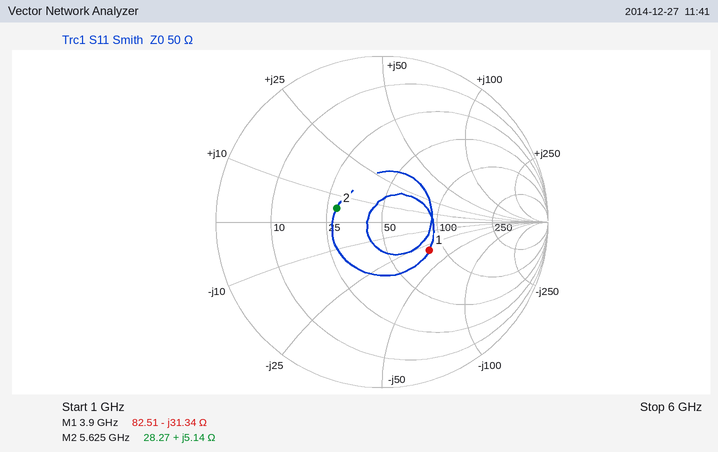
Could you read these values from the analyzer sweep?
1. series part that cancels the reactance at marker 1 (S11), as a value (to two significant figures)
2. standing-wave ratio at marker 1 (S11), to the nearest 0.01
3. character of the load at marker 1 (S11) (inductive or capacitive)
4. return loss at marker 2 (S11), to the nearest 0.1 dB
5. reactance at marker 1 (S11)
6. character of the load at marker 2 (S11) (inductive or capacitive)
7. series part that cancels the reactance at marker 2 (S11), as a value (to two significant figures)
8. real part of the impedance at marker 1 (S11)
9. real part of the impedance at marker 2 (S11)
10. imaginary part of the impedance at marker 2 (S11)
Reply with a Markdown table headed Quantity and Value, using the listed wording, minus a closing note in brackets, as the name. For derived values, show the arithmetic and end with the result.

| Quantity | Value |
|---|---|
| series part that cancels the reactance at marker 1 (S11), as a value | L = 31.34 Ω/(2π × 3.9 GHz) ≈ 1.3 nH |
| standing-wave ratio at marker 1 (S11), to the nearest 0.01 | 1.99 |
| character of the load at marker 1 (S11) | capacitive |
| return loss at marker 2 (S11), to the nearest 0.1 dB | 10.9 dB |
| reactance at marker 1 | -31.34 Ω |
| character of the load at marker 2 (S11) | inductive |
| series part that cancels the reactance at marker 2 (S11), as a value | C = 1/(2π × 5.625 GHz × 5.14 Ω) ≈ 5.5 pF |
| real part of the impedance at marker 1 | 82.51 Ω |
| real part of the impedance at marker 2 | 28.27 Ω |
| imaginary part of the impedance at marker 2 | +5.14 Ω |
